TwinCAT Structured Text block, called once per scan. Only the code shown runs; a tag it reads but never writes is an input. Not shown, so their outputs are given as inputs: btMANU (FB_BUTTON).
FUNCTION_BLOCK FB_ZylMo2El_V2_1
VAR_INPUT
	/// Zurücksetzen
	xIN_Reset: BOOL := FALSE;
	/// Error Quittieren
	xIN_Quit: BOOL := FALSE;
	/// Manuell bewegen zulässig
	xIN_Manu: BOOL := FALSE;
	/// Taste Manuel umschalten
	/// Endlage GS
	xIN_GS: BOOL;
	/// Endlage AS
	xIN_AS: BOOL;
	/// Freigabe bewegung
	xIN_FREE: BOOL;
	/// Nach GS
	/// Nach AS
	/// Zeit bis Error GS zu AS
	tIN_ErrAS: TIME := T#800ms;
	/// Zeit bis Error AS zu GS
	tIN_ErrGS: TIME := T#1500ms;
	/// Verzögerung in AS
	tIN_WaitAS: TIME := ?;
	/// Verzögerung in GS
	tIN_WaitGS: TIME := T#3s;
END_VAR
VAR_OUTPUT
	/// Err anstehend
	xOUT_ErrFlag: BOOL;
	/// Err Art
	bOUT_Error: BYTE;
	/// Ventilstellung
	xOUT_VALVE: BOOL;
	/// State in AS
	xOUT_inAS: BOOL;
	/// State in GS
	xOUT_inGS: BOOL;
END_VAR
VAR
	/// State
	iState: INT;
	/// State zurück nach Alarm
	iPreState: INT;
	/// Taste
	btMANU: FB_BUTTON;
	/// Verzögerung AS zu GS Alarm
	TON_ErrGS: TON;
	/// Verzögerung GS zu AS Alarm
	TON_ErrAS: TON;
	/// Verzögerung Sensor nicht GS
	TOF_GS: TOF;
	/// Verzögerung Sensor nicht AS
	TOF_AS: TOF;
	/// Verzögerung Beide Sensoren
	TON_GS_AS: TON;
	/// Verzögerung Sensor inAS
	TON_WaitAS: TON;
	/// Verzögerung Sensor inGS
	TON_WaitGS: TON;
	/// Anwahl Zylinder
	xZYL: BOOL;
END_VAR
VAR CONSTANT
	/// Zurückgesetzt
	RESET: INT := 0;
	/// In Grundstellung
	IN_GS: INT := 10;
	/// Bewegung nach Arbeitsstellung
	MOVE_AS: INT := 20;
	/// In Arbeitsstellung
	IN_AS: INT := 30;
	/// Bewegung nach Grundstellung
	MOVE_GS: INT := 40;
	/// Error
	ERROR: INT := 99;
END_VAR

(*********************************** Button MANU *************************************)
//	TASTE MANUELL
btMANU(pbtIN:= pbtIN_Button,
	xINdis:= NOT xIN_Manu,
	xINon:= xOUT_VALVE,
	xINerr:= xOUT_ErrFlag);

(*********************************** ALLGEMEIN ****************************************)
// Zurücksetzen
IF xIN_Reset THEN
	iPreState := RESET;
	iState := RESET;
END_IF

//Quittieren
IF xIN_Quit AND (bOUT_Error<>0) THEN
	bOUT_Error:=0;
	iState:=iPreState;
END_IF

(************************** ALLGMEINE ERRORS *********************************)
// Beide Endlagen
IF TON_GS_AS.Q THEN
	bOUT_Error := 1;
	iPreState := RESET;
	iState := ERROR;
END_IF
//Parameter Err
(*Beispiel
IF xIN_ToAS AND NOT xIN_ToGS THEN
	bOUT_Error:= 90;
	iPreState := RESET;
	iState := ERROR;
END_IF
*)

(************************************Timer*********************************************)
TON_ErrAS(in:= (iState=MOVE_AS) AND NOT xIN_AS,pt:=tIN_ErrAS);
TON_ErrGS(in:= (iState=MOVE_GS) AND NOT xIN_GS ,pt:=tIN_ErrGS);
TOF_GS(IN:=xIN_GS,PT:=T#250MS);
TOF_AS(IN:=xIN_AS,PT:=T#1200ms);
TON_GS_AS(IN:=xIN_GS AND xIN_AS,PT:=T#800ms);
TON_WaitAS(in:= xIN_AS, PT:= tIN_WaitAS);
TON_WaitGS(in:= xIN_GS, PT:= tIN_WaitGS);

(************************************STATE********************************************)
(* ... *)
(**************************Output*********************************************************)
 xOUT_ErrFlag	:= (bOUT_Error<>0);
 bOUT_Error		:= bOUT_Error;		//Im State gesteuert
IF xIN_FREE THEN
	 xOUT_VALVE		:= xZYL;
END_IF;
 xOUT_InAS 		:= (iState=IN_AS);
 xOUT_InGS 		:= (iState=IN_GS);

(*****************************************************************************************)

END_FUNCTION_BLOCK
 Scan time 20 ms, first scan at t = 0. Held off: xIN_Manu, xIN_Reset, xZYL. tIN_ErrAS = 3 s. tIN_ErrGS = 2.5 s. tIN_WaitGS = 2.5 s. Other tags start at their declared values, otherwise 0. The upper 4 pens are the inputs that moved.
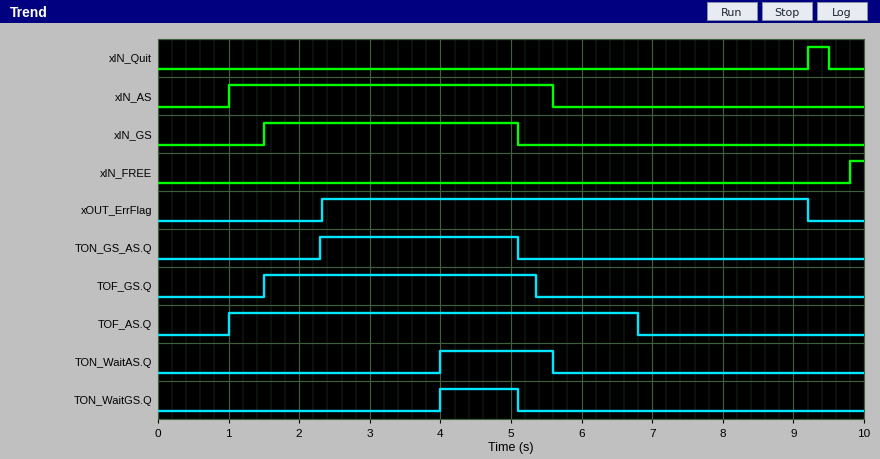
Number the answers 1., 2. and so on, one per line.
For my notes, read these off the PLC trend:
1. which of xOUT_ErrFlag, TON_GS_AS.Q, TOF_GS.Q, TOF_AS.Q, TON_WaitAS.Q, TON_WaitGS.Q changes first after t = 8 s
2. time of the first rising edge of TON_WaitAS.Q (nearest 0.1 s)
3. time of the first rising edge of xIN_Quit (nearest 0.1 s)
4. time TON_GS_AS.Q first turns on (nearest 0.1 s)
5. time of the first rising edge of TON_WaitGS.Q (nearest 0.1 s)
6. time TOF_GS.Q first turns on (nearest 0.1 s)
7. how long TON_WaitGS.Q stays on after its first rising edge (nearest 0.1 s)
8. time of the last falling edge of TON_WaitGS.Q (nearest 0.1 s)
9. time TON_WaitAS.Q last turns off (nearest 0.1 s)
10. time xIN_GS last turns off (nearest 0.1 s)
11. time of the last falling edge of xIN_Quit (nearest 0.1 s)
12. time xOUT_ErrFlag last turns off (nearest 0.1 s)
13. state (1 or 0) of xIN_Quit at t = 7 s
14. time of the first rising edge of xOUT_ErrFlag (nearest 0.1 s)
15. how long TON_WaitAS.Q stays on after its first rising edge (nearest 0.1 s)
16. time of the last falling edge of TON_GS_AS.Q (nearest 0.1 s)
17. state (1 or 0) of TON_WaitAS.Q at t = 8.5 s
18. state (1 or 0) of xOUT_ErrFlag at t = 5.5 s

1. xOUT_ErrFlag
2. 4.0 s
3. 9.2 s
4. 2.3 s
5. 4.0 s
6. 1.5 s
7. 1.1 s
8. 5.1 s
9. 5.6 s
10. 5.1 s
11. 9.5 s
12. 9.2 s
13. 0
14. 2.3 s
15. 1.6 s
16. 5.1 s
17. 0
18. 1
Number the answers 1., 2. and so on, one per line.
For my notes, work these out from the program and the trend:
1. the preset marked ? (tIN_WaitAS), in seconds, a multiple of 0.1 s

1. 3.0 s
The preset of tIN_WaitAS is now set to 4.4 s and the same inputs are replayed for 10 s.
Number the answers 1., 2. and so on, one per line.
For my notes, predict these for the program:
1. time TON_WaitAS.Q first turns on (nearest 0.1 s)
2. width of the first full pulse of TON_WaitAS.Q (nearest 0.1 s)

1. 5.4 s
2. 0.2 s
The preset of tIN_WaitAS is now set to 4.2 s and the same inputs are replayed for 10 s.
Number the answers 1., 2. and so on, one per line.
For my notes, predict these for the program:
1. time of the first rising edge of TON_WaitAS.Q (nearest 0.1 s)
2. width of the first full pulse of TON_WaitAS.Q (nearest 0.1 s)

1. 5.2 s
2. 0.4 s
